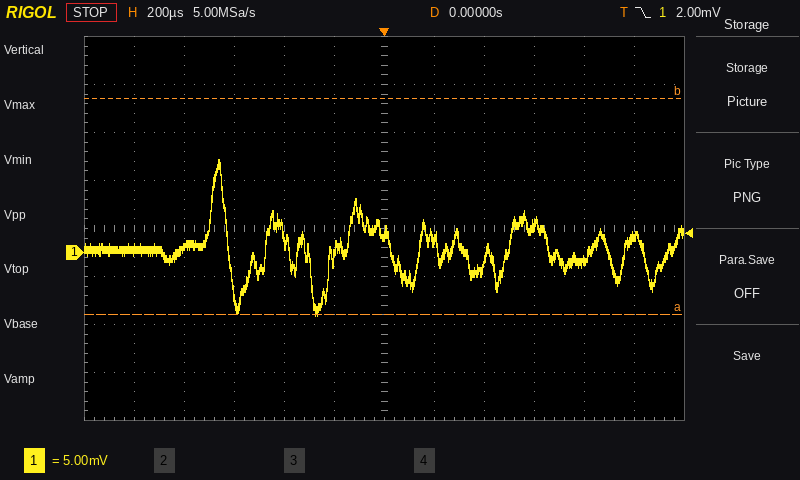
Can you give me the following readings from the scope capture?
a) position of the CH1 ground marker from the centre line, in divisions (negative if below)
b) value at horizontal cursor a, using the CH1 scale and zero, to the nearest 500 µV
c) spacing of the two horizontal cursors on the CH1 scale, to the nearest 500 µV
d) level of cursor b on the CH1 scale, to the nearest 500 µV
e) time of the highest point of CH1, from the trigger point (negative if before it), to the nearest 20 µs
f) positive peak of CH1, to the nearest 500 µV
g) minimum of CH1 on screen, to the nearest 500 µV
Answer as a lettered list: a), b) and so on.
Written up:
a) -0.5 div
b) -6.5 mV
c) 22.5 mV
d) 16.0 mV
e) -660 µs
f) 9.5 mV
g) -6.5 mV
